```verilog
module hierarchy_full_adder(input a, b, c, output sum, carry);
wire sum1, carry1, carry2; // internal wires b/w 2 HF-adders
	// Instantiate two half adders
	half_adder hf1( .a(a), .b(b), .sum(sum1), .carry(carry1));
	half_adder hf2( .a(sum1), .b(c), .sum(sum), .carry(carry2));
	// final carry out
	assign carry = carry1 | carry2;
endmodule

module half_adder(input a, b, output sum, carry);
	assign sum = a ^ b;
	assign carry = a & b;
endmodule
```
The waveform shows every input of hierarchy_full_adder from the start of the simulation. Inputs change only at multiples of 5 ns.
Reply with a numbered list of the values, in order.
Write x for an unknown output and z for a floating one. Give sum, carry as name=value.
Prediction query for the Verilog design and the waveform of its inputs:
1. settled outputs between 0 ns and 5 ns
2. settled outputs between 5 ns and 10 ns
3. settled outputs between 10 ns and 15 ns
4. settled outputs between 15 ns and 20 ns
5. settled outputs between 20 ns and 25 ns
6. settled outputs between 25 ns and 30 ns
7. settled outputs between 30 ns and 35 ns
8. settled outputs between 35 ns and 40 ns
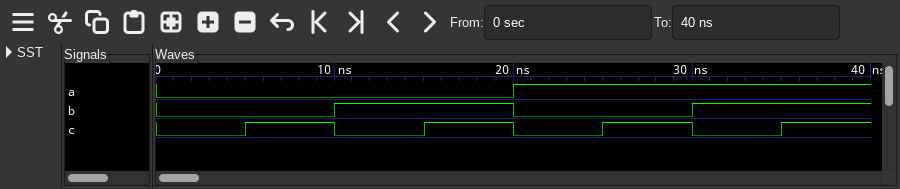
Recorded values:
1. sum=0, carry=0
2. sum=1, carry=0
3. sum=1, carry=0
4. sum=0, carry=1
5. sum=1, carry=0
6. sum=0, carry=1
7. sum=0, carry=1
8. sum=1, carry=1
